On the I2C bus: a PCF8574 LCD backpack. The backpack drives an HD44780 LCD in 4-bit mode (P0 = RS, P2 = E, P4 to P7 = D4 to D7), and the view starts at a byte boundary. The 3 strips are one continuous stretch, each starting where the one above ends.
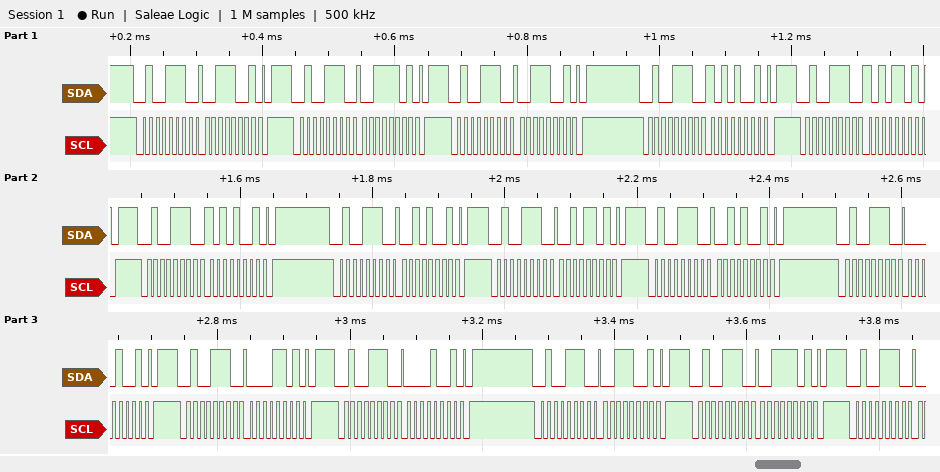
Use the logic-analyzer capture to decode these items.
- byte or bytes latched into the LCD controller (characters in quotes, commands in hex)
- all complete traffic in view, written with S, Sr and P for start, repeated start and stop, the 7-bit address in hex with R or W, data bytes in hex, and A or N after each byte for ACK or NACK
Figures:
':' ' '
S 27W A 39 A P S 27W A 3D A P S 27W A 39 A P S 27W A A9 A P S 27W A AD A P S 27W A A9 A P S 27W A 29 A P S 27W A 2D A P S 27W A 29 A P S 27W A 09 A P S 27W A 0D A P S 27W A 09 A P S 27W A 39 A P S 27W A 3D A P S 27W A
